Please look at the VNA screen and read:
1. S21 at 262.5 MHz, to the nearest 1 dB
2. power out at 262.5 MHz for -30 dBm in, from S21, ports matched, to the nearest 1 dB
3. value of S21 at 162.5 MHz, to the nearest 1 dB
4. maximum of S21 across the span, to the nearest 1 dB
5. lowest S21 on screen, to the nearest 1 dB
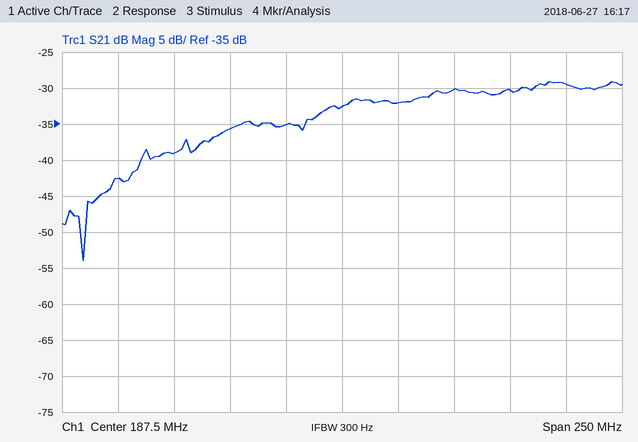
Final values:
-30 dB
-60 dBm
-35 dB
-29 dB
-54 dB
